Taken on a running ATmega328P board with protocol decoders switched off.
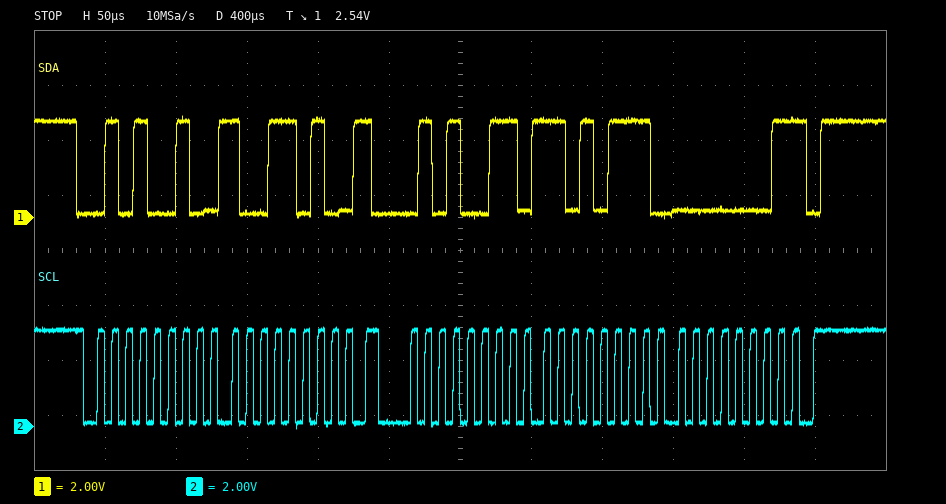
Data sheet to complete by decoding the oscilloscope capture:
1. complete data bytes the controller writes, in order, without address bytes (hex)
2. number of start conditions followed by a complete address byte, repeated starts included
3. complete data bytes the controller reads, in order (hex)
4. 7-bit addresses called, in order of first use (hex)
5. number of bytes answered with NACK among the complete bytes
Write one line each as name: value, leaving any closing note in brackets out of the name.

complete data bytes the controller writes, in order, without address bytes: 9A
number of start conditions followed by a complete address byte, repeated starts included: 2
complete data bytes the controller reads, in order: D7 01
7-bit addresses called, in order of first use: 0x29
number of bytes answered with NACK among the complete bytes: 1
